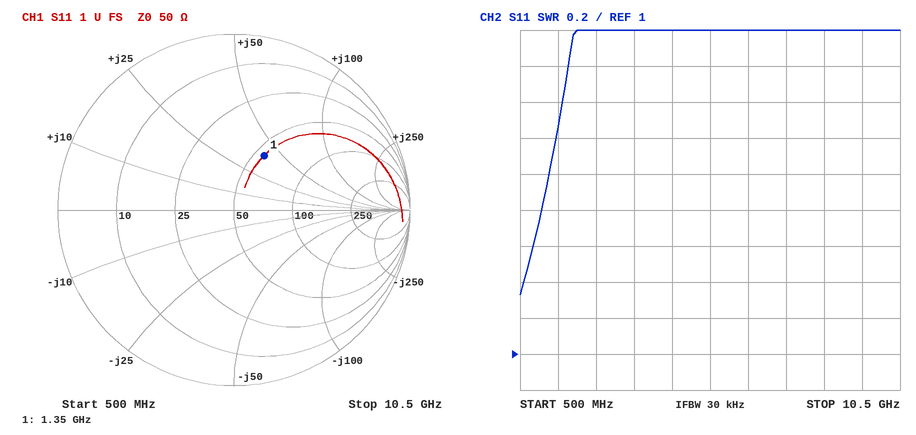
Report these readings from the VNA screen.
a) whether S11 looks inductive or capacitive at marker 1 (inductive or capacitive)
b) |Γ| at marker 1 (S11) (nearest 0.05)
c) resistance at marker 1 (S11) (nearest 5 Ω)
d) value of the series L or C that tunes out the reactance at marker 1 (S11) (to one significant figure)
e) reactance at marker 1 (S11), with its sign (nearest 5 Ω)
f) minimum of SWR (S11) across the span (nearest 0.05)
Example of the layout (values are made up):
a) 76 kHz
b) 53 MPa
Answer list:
a) inductive
b) 0.35
c) 55 Ω
d) 3 pF
e) +40 Ω
f) 1.35
